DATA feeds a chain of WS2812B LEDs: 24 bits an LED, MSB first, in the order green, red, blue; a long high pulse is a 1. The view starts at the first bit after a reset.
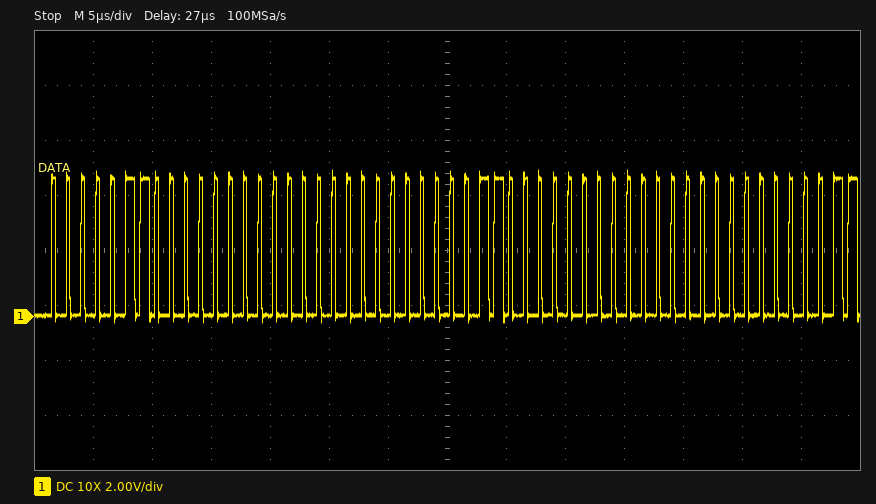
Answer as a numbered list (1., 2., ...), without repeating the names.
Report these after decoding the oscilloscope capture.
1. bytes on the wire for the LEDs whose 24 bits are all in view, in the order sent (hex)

1. 06 00 00 06 00 00
